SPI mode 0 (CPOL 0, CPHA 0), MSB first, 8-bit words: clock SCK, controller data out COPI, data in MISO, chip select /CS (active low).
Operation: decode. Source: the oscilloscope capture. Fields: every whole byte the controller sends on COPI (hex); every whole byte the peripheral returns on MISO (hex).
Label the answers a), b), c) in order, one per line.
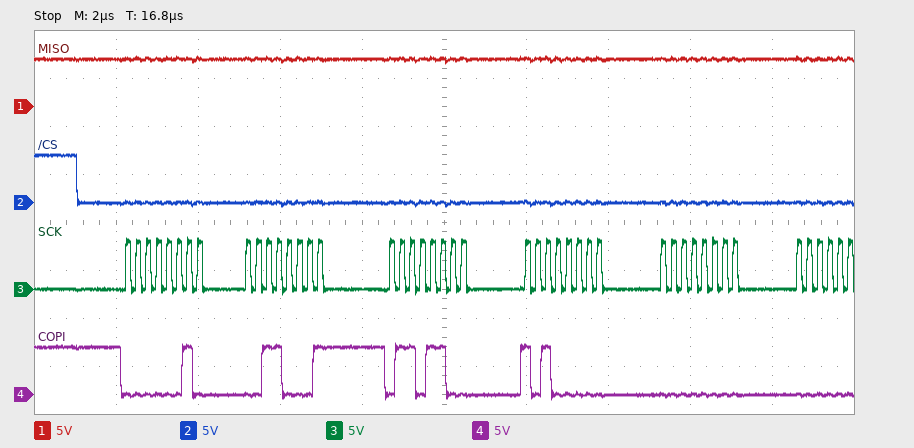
a) 0x02 0x31 0x6C 0xA0 0x00
b) 0xFF 0xFF 0xFF 0xFF 0xFF
